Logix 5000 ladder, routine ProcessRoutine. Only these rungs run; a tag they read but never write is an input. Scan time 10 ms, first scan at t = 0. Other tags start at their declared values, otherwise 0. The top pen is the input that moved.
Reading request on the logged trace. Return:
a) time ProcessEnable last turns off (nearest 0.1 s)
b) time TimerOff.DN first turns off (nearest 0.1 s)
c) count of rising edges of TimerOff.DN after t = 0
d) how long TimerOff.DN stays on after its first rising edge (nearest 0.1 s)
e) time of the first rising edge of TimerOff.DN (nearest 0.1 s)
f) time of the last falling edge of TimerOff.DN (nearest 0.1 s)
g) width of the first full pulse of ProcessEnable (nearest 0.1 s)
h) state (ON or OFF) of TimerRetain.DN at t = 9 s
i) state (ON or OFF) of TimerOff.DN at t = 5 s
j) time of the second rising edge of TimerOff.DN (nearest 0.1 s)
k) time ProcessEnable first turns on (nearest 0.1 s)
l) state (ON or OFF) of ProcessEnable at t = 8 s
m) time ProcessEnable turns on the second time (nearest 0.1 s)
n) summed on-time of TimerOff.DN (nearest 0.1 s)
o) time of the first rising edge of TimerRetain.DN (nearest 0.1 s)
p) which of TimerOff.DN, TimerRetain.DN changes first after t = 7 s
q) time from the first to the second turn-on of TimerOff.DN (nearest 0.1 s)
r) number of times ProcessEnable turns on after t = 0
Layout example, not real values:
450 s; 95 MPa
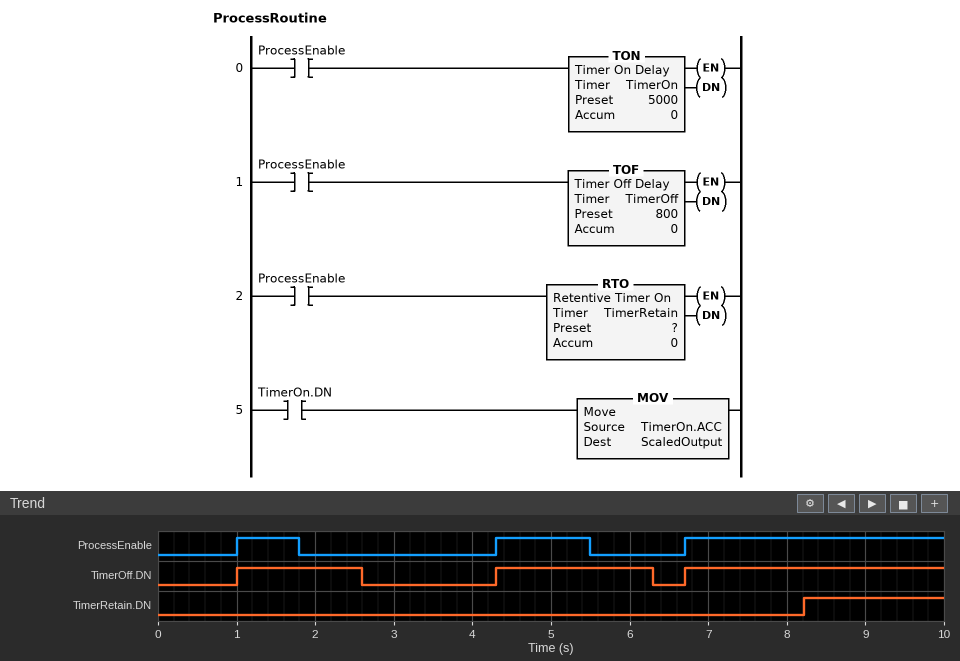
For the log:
5.5 s; 2.6 s; 3; 1.6 s; 1.0 s; 6.3 s; 0.8 s; ON; ON; 4.3 s; 1.0 s; ON; 4.3 s; 6.9 s; 8.2 s; TimerRetain.DN; 3.3 s; 3
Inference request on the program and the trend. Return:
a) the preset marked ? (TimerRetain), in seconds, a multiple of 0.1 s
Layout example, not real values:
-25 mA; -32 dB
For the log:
3.5 s
